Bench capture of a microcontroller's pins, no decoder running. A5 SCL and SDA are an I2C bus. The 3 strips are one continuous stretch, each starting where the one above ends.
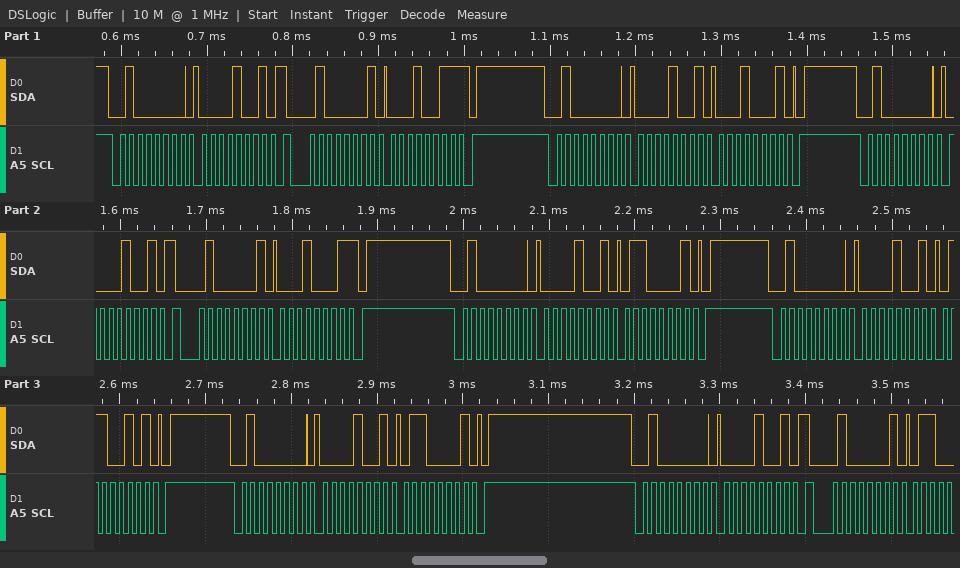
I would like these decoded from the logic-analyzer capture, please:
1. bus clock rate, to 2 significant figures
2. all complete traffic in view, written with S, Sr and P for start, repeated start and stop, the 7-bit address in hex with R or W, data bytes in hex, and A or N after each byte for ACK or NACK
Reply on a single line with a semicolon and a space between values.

100 kHz; S 20W A 09 A Sr 20R A 13 N P S 20W A 09 A 11 A P S 20W A 09 A Sr 20R A 11 N P S 20W A 09 A 61 A P S 20W A 09 A 65 A P S 20W A 09 A 61 A P S 20W A 09 A Sr 20R A
